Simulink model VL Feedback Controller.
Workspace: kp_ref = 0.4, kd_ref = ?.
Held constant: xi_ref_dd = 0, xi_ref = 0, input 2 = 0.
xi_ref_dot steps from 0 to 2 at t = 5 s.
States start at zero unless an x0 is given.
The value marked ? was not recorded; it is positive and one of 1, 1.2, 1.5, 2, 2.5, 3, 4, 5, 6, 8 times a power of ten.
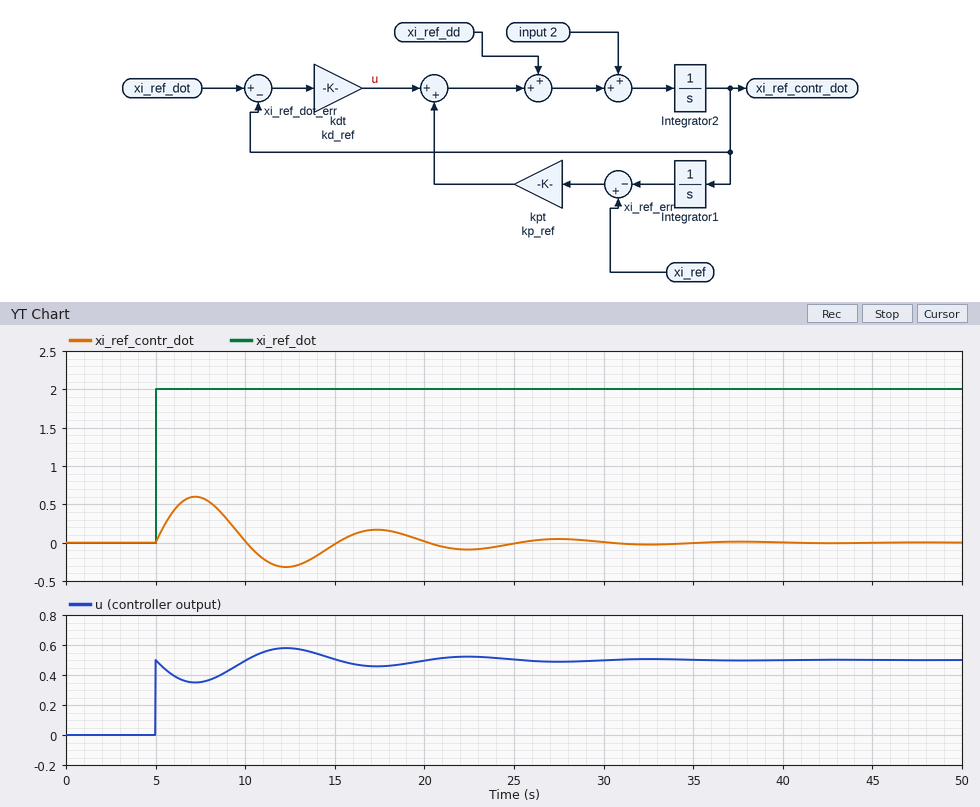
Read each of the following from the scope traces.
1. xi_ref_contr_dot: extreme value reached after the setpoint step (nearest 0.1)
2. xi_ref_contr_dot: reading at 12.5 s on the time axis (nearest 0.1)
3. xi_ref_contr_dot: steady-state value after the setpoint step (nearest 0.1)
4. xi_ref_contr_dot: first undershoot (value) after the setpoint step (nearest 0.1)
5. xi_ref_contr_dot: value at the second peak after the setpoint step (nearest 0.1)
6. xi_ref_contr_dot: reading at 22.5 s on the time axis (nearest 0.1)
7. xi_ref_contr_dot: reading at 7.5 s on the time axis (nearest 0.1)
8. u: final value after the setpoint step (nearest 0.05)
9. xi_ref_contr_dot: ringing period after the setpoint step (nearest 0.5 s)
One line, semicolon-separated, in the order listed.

0.6; -0.3; 0.0; -0.3; 0.2; -0.1; 0.6; 0.50; 10.0 s
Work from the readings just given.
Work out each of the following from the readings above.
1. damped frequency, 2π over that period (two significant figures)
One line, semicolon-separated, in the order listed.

0.63 rad/s
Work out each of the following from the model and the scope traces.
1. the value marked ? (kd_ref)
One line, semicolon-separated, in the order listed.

0.25
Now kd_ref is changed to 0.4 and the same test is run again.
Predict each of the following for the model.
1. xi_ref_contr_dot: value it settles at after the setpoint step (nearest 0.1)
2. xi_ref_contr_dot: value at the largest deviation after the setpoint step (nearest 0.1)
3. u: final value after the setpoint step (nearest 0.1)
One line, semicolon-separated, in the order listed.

0.0; 0.8; 0.8
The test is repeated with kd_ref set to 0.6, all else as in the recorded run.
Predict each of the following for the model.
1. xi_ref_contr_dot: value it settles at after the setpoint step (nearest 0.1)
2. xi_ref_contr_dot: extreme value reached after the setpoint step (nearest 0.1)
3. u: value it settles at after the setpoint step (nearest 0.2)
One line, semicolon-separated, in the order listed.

0.0; 1.1; 1.2
